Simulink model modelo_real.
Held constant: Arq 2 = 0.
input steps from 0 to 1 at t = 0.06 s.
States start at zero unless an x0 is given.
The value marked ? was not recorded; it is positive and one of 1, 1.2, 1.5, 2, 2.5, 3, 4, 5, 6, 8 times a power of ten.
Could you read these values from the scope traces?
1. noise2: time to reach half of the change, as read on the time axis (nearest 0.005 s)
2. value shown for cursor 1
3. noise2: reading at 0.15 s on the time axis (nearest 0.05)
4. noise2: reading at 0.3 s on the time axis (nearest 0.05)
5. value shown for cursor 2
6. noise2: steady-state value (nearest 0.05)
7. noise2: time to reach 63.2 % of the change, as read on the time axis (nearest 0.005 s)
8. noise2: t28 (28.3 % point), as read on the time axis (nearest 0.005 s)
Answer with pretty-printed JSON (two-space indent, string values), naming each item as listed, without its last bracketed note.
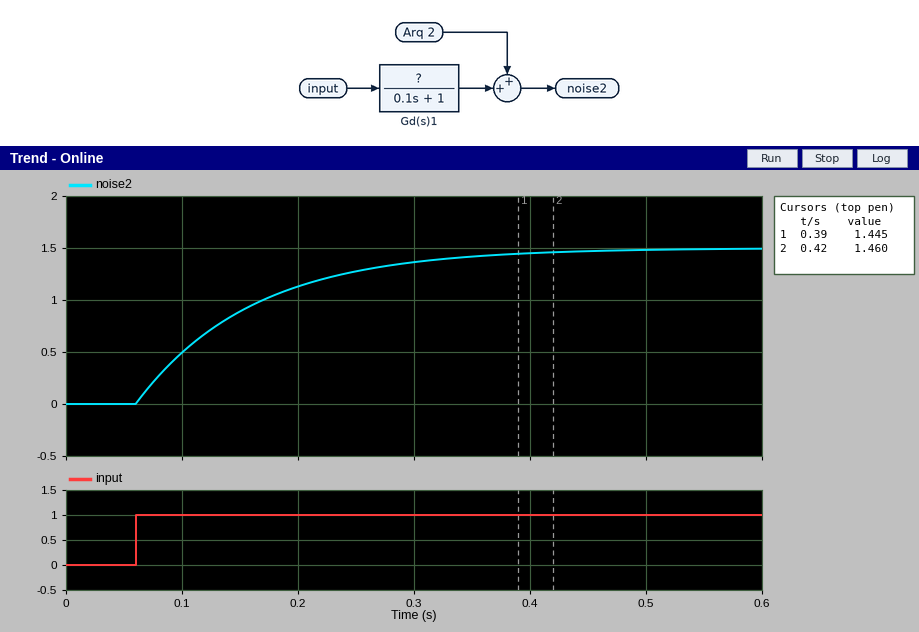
{
  "noise2: time to reach half of the change, as read on the time axis": "0.130 s",
  "value shown for cursor 1": "1.445",
  "noise2: reading at 0.15 s on the time axis": "0.90",
  "noise2: reading at 0.3 s on the time axis": "1.35",
  "value shown for cursor 2": "1.460",
  "noise2: steady-state value": "1.50",
  "noise2: time to reach 63.2 % of the change, as read on the time axis": "0.160 s",
  "noise2: t28 (28.3 % point), as read on the time axis": "0.095 s"
}
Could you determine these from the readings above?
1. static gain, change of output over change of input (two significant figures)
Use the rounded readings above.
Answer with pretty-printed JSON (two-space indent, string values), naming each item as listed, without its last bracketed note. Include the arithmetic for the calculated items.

{
  "static gain, change of output over change of input": "(1.5 - 0) / (1 - 0) = 1.5"
}
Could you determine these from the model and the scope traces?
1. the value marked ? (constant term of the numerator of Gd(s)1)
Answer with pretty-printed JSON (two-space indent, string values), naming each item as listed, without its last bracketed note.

{
  "the value marked ? (constant term of the numerator of Gd(s)1)": "1.5"
}
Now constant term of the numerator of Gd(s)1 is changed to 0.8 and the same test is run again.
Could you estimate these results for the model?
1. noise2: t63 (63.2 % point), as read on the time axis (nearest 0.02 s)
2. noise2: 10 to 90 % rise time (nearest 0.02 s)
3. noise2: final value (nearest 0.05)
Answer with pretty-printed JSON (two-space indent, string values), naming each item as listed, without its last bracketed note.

{
  "noise2: t63 (63.2 % point), as read on the time axis": "0.16 s",
  "noise2: 10 to 90 % rise time": "0.22 s",
  "noise2: final value": "0.80"
}
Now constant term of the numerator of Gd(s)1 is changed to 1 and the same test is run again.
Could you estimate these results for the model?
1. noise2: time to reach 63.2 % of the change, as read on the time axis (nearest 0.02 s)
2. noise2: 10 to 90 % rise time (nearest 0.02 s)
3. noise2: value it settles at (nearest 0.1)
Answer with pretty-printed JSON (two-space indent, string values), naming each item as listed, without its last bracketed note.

{
  "noise2: time to reach 63.2 % of the change, as read on the time axis": "0.16 s",
  "noise2: 10 to 90 % rise time": "0.22 s",
  "noise2: value it settles at": "1.0"
}
